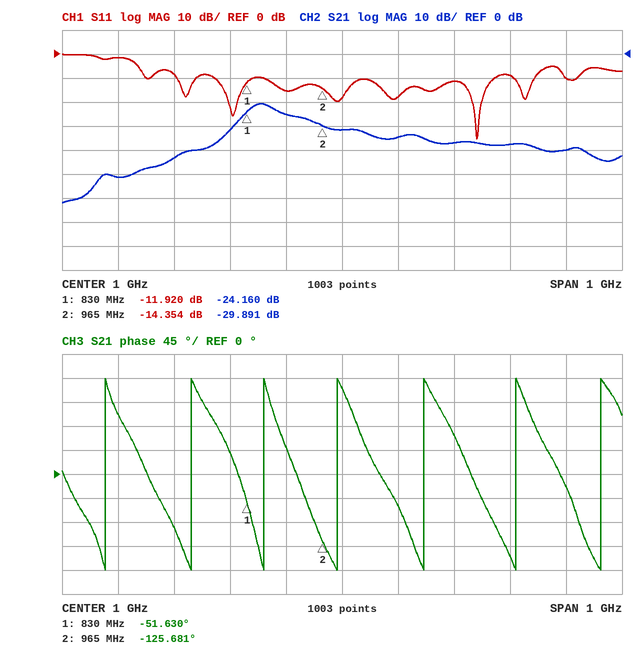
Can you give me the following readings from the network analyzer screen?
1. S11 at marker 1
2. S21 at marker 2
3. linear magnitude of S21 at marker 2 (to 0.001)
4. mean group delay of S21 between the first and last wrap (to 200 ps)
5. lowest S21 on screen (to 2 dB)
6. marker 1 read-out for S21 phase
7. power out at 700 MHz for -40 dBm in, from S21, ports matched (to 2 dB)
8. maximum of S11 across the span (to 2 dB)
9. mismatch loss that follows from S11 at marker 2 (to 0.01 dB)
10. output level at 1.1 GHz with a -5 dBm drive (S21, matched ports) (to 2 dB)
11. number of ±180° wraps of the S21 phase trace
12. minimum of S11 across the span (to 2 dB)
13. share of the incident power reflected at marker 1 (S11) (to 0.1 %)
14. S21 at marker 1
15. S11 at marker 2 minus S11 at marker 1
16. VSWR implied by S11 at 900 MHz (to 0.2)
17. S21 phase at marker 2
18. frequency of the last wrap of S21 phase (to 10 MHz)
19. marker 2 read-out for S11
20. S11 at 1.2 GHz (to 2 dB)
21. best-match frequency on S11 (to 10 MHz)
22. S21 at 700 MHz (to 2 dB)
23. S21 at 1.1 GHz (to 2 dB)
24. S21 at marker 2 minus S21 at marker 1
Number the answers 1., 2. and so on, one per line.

1. -11.920 dB
2. -29.891 dB
3. 0.032
4. 6.8 ns
5. -62 dB
6. -51.630°
7. -84 dBm
8. 0 dB
9. 0.16 dB
10. -40 dBm
11. 7
12. -36 dB
13. 6.4 %
14. -24.160 dB
15. -2.434 dB
16. 1.4
17. -125.681°
18. 1.46 GHz
19. -14.354 dB
20. -12 dB
21. 1.24 GHz
22. -44 dB
23. -34 dB
24. -5.731 dB
